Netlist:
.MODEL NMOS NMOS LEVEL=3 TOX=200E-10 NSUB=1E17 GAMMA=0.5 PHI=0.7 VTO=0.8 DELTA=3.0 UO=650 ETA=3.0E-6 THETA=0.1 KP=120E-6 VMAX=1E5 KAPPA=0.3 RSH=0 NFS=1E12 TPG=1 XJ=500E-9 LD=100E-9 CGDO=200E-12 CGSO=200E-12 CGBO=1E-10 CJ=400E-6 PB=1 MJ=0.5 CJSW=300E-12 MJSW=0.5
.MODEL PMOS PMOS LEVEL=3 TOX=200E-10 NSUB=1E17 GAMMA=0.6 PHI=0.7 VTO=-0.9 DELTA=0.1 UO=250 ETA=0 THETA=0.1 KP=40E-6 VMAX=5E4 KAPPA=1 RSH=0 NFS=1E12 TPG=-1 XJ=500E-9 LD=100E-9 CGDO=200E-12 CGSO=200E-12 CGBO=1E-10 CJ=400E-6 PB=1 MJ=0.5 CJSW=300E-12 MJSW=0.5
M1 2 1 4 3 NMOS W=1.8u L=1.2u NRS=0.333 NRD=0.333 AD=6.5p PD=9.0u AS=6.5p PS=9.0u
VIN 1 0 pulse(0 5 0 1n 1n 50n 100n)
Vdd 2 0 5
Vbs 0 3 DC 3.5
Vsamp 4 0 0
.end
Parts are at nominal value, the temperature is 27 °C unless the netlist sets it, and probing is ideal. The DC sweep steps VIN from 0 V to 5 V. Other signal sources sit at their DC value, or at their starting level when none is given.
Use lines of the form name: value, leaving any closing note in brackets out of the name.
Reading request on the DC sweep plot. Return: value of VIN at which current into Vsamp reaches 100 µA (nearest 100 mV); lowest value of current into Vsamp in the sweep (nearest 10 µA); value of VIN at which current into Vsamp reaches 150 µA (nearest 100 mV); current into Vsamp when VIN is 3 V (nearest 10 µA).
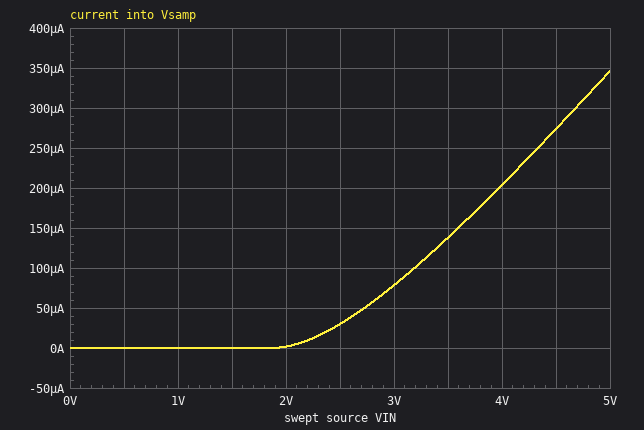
value of VIN at which current into Vsamp reaches 100 µA: 3.2 V
lowest value of current into Vsamp in the sweep: 0 A
value of VIN at which current into Vsamp reaches 150 µA: 3.6 V
current into Vsamp when VIN is 3 V: 80 µA
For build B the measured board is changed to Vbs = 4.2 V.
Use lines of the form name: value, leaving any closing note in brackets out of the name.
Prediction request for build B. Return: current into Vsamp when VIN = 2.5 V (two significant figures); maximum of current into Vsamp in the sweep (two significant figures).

current into Vsamp when VIN = 2.5 V: 18 µA
maximum of current into Vsamp in the sweep: 320 µA
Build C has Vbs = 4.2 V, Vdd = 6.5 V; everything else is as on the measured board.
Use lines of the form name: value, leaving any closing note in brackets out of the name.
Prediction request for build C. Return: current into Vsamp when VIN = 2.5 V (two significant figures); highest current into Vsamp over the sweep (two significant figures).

current into Vsamp when VIN = 2.5 V: 18 µA
highest current into Vsamp over the sweep: 330 µA
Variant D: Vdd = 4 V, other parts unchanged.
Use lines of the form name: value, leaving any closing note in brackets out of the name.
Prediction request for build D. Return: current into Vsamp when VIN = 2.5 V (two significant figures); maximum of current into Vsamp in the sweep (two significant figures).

current into Vsamp when VIN = 2.5 V: 29 µA
maximum of current into Vsamp in the sweep: 340 µA
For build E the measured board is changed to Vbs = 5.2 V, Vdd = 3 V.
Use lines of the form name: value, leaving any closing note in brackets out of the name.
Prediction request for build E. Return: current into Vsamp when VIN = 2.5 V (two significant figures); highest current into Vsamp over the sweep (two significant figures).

current into Vsamp when VIN = 2.5 V: 5.5 µA
highest current into Vsamp over the sweep: 280 µA
